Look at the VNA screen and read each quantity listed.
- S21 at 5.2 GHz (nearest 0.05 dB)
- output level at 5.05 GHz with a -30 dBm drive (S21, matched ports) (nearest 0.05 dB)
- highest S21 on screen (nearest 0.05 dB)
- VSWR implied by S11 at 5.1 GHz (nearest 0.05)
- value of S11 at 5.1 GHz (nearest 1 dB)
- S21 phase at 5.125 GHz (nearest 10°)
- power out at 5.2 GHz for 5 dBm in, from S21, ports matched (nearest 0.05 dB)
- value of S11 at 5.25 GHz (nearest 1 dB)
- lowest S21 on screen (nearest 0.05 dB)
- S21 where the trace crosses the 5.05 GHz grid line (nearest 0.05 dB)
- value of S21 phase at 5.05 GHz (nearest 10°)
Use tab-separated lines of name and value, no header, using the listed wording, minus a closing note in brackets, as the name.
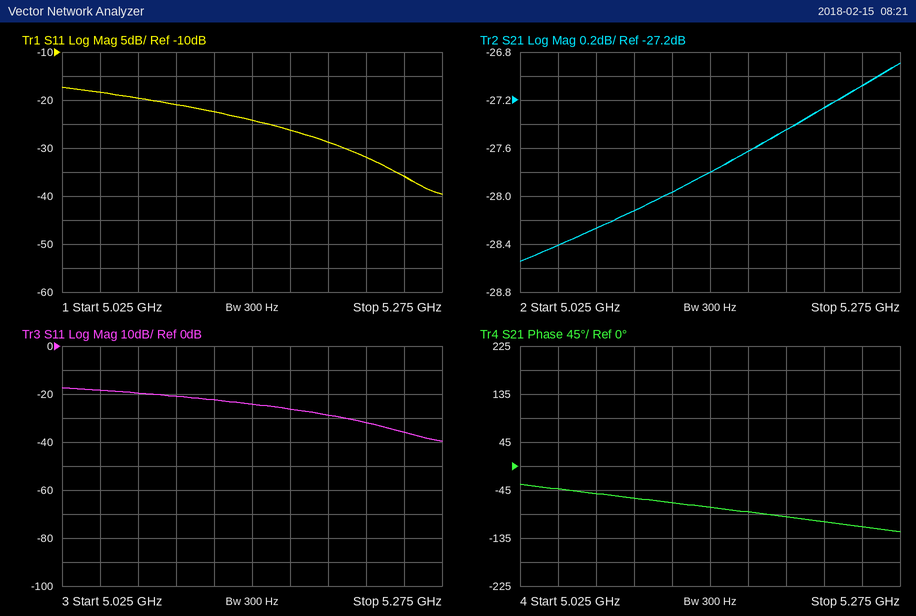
S21 at 5.2 GHz	-27.45 dB
output level at 5.05 GHz with a -30 dBm drive (S21, matched ports)	-58.40 dBm
highest S21 on screen	-26.90 dB
VSWR implied by S11 at 5.1 GHz	1.20
value of S11 at 5.1 GHz	-21 dB
S21 phase at 5.125 GHz	-70°
power out at 5.2 GHz for 5 dBm in, from S21, ports matched	-22.45 dBm
value of S11 at 5.25 GHz	-36 dB
lowest S21 on screen	-28.55 dB
S21 where the trace crosses the 5.05 GHz grid line	-28.40 dB
value of S21 phase at 5.05 GHz	-40°
